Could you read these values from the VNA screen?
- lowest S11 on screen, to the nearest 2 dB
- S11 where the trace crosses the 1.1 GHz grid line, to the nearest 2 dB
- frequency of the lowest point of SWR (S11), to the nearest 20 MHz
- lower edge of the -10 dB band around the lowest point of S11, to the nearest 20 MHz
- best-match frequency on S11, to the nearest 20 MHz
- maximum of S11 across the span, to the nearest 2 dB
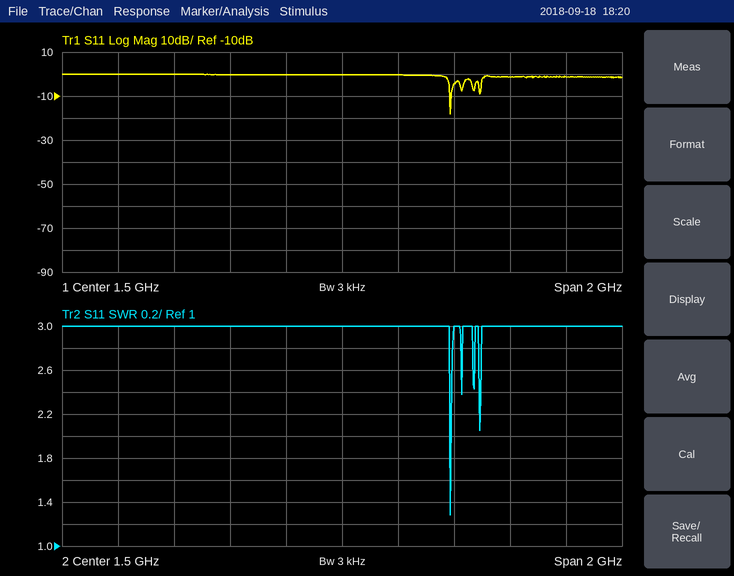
-18 dB
0 dB
1.88 GHz
1.88 GHz
1.88 GHz
0 dB
